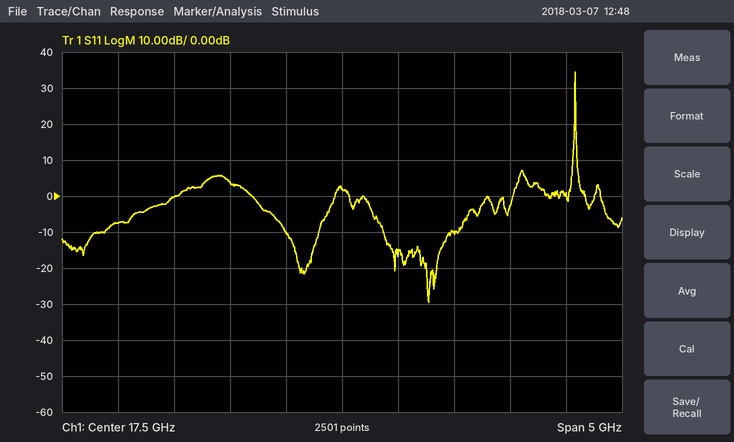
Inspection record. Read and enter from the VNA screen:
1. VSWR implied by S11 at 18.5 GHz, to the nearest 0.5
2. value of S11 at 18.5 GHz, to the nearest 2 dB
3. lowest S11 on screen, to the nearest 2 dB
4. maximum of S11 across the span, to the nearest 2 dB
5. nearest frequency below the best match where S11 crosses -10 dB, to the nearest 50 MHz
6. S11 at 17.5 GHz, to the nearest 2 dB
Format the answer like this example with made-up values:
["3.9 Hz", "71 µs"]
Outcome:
["2.0", "-10 dB", "-30 dB", "34 dB", "17.85 GHz", "2 dB"]
